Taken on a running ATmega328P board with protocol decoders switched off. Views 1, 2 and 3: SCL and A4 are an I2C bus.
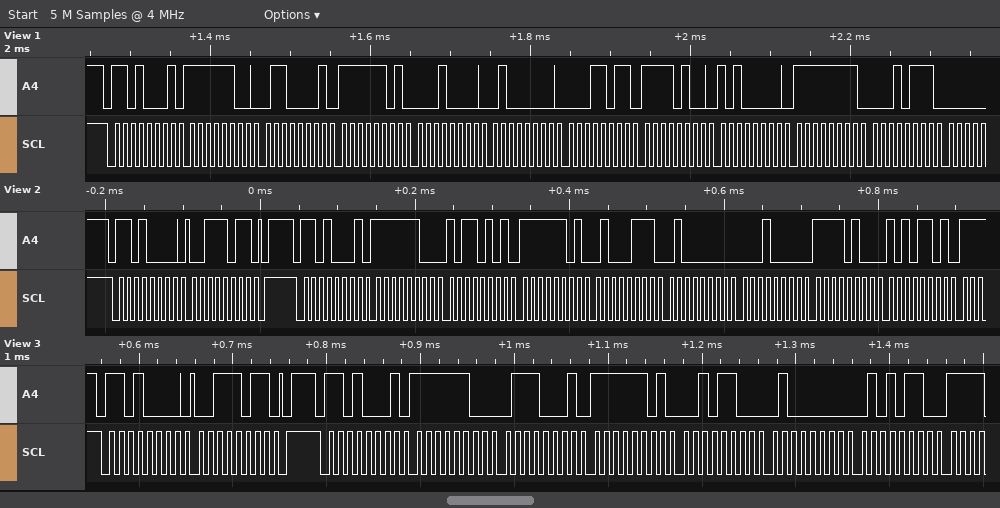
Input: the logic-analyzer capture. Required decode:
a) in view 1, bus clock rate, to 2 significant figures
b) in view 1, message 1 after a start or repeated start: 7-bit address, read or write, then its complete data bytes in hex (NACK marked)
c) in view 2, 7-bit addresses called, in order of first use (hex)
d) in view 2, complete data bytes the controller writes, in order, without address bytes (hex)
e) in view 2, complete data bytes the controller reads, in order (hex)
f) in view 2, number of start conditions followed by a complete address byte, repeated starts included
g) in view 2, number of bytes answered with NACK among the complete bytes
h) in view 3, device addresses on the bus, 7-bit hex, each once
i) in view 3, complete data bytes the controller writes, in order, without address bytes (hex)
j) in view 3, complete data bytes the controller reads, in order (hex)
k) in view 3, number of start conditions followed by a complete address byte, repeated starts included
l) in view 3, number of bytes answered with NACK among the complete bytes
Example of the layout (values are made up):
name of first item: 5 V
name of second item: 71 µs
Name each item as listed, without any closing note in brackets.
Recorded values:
in view 1, bus clock rate, to 2 significant figures: 100 kHz
in view 1, message 1 after a start or repeated start: 7-bit address, read or write, then its complete data bytes in hex: 0x68 read: FC 61 FD 10 40 1B F4 A0 FF 17
in view 2, 7-bit addresses called, in order of first use: 0x68
in view 2, complete data bytes the controller writes, in order, without address bytes: 3B
in view 2, complete data bytes the controller reads, in order: FC B5 FD 47 40 10 F4 AD
in view 2, number of start conditions followed by a complete address byte, repeated starts included: 2
in view 2, number of bytes answered with NACK among the complete bytes: 0
in view 3, device addresses on the bus, 7-bit hex, each once: 0x68
in view 3, complete data bytes the controller writes, in order, without address bytes: 3B
in view 3, complete data bytes the controller reads, in order: FC 71 FD 2C 40 56
in view 3, number of start conditions followed by a complete address byte, repeated starts included: 2
in view 3, number of bytes answered with NACK among the complete bytes: 0
